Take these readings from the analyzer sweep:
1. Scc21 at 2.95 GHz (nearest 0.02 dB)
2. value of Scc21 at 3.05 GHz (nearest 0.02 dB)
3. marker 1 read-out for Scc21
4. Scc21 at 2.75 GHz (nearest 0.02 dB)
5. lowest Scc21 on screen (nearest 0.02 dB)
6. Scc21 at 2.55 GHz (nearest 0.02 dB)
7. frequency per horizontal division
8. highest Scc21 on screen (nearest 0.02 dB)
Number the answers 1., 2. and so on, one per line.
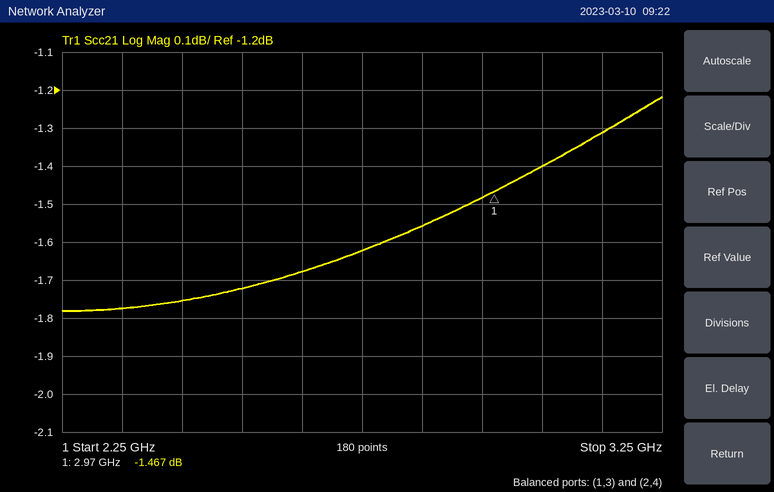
1. -1.48 dB
2. -1.40 dB
3. -1.467 dB
4. -1.62 dB
5. -1.78 dB
6. -1.72 dB
7. 100 MHz
8. -1.22 dB
